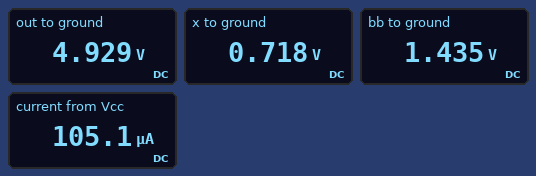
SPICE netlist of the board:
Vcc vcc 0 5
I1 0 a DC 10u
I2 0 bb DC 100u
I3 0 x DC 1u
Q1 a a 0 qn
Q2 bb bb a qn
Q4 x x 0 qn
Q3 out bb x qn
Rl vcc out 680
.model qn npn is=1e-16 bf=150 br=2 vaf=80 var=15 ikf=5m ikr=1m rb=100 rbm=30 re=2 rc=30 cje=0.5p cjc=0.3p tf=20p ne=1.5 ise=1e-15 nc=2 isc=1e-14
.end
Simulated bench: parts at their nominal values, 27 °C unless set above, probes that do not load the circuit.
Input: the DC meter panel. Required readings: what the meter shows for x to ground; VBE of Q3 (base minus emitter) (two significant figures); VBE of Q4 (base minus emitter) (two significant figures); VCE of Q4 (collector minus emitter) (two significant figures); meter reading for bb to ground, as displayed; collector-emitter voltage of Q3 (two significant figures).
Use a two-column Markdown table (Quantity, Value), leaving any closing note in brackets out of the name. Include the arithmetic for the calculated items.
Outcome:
| Quantity | Value |
|---|---|
| what the meter shows for x to ground | 0.718 V |
| VBE of Q3 (base minus emitter) | 1.435 V - 718 mV = 720 mV |
| VBE of Q4 (base minus emitter) | 718 mV = 720 mV |
| VCE of Q4 (collector minus emitter) | 718 mV = 720 mV |
| meter reading for bb to ground, as displayed | 1.435 V |
| collector-emitter voltage of Q3 | 4.929 V - 718 mV = 4.2 V |
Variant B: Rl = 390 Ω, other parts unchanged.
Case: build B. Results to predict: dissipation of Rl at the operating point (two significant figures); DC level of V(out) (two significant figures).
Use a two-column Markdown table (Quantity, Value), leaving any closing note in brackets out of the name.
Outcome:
| Quantity | Value |
|---|---|
| dissipation of Rl at the operating point | 4.3 µW |
| DC level of V(out) | 5.0 V |
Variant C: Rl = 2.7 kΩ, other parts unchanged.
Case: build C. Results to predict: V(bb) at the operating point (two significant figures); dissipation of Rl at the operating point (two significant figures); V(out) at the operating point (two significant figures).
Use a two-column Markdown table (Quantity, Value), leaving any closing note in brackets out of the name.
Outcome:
| Quantity | Value |
|---|---|
| V(bb) at the operating point | 1.4 V |
| dissipation of Rl at the operating point | 30 µW |
| V(out) at the operating point | 4.7 V |
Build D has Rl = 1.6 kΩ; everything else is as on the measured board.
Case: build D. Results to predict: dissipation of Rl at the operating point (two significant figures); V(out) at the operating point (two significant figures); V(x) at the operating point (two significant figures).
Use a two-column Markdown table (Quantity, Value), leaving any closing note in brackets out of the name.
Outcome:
| Quantity | Value |
|---|---|
| dissipation of Rl at the operating point | 18 µW |
| V(out) at the operating point | 4.8 V |
| V(x) at the operating point | 720 mV |
